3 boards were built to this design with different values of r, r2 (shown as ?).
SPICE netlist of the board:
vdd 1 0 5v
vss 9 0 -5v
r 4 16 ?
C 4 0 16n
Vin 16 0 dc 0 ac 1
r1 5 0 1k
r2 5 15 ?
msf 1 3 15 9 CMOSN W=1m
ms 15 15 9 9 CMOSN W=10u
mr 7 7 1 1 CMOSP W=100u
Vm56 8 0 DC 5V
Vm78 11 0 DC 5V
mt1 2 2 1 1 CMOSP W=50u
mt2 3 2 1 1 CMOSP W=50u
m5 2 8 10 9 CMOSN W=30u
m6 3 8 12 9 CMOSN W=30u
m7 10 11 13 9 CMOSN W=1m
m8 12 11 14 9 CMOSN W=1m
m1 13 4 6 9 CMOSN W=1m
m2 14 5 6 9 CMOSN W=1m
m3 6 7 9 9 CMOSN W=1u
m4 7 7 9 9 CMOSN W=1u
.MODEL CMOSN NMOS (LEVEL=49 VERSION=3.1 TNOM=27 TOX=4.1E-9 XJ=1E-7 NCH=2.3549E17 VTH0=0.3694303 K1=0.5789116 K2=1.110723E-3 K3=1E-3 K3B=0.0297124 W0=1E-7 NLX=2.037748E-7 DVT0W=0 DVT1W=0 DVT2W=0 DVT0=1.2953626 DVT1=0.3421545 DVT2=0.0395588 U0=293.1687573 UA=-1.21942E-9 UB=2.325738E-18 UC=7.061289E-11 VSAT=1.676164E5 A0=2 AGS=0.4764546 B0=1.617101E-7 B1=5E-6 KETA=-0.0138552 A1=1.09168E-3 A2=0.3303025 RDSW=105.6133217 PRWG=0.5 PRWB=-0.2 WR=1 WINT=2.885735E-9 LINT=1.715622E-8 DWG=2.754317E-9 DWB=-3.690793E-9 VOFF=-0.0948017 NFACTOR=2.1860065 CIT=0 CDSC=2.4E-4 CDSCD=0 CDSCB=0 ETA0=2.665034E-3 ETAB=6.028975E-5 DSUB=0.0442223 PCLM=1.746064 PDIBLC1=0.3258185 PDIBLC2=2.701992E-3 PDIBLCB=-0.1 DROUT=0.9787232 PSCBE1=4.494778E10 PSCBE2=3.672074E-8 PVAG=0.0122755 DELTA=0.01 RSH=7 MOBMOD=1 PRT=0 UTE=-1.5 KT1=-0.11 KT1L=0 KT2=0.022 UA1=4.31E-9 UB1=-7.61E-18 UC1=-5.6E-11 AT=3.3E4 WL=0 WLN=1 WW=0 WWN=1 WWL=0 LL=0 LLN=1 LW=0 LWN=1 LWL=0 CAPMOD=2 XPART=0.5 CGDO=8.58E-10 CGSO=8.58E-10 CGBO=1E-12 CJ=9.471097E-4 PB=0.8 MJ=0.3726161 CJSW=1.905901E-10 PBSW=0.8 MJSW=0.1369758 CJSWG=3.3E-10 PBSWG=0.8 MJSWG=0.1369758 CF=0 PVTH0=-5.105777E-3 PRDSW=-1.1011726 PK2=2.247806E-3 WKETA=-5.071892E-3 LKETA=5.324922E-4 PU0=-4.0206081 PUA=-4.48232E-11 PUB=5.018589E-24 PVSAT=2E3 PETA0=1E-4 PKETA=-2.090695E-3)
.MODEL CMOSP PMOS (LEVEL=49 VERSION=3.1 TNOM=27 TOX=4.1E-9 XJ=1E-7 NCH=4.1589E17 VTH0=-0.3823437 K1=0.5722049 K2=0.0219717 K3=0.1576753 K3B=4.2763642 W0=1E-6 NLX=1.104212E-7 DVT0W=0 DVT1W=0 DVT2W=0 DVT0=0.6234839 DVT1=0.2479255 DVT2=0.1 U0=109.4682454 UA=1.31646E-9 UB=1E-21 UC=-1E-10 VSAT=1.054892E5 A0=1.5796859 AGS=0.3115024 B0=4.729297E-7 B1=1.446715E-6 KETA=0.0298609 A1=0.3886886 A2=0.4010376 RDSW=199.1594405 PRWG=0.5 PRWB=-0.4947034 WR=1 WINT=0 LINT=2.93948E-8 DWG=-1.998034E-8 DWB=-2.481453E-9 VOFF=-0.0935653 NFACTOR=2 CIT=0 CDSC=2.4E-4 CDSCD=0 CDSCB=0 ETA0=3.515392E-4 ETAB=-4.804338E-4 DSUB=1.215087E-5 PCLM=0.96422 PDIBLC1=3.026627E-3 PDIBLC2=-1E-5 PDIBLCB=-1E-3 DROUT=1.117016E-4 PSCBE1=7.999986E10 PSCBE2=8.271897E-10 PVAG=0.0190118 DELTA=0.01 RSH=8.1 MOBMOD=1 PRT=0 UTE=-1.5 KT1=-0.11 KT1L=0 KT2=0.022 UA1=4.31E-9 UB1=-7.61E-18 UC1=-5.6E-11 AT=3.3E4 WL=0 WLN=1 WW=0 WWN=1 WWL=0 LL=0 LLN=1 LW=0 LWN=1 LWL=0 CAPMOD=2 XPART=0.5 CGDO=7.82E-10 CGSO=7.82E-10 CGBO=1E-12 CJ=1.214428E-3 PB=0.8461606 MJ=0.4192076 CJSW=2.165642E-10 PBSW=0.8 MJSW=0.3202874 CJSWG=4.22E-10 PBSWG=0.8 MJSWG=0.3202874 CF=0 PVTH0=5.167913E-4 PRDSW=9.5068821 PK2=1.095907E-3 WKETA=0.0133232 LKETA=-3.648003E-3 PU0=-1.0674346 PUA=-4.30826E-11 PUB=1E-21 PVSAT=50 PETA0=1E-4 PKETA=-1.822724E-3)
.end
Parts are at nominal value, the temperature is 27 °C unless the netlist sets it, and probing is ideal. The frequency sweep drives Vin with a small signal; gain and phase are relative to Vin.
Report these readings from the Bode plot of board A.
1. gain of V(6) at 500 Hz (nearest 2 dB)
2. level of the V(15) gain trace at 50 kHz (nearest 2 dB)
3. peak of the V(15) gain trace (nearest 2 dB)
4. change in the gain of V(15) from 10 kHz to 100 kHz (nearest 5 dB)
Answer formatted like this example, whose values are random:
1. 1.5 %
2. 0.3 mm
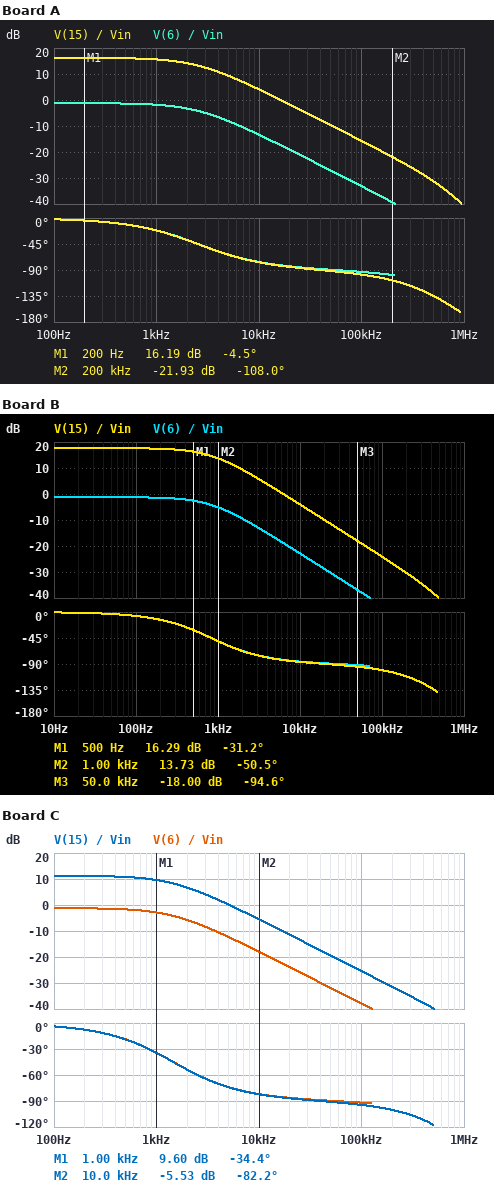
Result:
1. -2 dB
2. -10 dB
3. 16 dB
4. -20 dB
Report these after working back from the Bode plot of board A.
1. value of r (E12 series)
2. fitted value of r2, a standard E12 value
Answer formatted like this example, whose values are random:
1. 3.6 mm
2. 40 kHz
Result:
1. 3.9 kΩ
2. 5.6 kΩ
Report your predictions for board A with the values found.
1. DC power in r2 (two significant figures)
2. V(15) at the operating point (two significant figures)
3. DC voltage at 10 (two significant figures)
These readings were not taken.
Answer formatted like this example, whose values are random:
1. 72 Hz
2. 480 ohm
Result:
1. 120 nW
2. 31 mV
3. 3.1 V
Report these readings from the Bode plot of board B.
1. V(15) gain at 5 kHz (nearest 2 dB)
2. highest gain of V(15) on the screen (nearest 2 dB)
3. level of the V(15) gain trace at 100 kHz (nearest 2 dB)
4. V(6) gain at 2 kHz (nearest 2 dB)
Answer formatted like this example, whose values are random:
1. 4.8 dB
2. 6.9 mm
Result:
1. 2 dB
2. 18 dB
3. -24 dB
4. -10 dB
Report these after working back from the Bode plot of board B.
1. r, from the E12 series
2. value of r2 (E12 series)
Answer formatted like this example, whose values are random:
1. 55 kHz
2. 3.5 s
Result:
1. 12 kΩ
2. 6.8 kΩ
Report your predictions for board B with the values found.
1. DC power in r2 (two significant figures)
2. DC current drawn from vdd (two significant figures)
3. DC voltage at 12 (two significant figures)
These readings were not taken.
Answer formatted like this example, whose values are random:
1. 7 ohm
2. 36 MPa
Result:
1. 150 nW
2. 3.1 mA
3. 1.6 V
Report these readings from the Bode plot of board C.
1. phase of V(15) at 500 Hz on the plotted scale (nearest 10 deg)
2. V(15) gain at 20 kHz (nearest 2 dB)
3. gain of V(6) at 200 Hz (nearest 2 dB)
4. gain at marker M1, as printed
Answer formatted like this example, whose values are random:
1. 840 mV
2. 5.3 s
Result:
1. -20 deg
2. -12 dB
3. -2 dB
4. 9.60 dB
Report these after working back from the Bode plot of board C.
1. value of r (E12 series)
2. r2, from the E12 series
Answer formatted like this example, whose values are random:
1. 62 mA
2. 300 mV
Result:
1. 6.8 kΩ
2. 2.7 kΩ
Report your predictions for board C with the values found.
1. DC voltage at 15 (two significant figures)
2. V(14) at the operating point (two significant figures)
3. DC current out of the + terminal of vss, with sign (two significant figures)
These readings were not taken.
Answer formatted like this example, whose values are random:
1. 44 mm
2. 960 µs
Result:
1. 17 mV
2. 1.5 V
3. -3.0 mA
